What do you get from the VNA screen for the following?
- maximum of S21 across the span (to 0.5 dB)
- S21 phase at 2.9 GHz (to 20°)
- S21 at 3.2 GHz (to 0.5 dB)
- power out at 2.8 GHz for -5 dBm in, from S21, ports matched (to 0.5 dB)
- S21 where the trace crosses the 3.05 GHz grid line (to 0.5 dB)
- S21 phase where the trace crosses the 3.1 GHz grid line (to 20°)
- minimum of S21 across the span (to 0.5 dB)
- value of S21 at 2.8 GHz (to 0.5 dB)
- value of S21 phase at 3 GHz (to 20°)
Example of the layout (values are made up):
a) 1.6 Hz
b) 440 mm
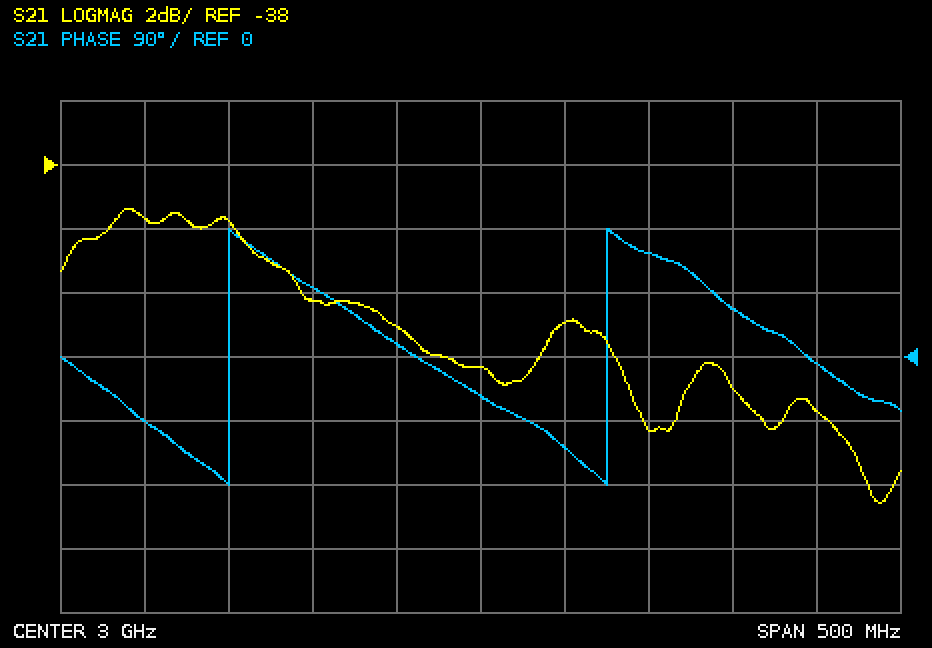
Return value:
a) -39.5 dB
b) 100°
c) -45.5 dB
d) -44.5 dBm
e) -43.0 dB
f) 140°
g) -48.5 dB
h) -39.5 dB
i) -60°
